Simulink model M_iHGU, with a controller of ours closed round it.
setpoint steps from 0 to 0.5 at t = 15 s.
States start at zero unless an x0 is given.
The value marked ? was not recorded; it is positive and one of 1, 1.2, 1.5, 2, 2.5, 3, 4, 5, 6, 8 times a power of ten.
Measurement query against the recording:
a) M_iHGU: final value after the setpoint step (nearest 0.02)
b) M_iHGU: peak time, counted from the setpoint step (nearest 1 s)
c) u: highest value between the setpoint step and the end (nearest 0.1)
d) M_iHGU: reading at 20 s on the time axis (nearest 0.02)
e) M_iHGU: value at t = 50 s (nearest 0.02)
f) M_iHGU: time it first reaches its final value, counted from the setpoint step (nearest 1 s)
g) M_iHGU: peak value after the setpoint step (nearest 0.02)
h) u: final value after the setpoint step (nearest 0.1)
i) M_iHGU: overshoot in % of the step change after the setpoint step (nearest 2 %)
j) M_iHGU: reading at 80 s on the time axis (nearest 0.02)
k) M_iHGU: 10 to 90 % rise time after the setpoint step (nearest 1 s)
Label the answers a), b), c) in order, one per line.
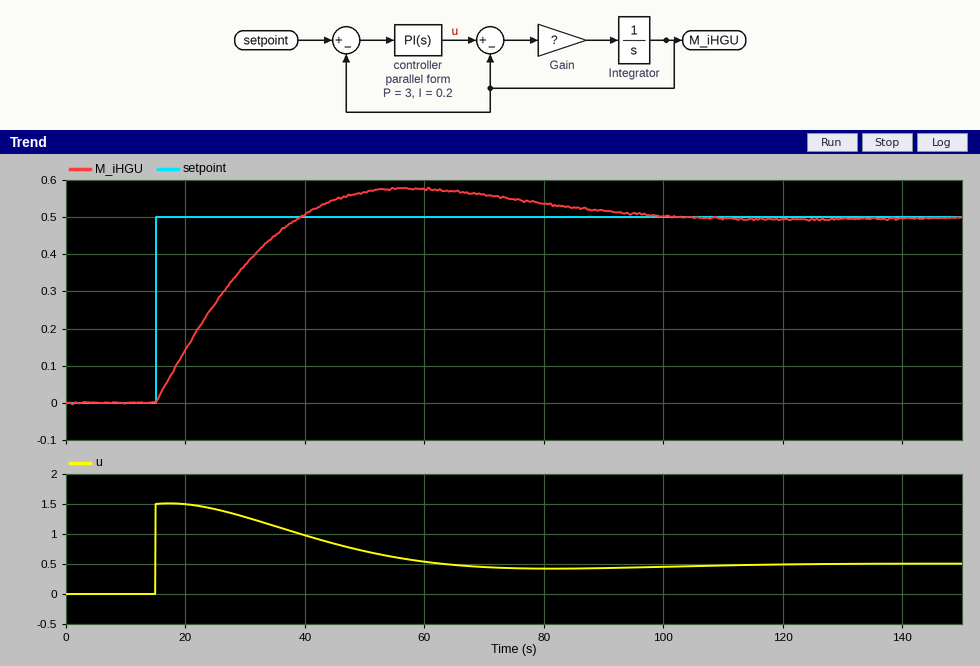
a) 0.50
b) 42 s
c) 1.5
d) 0.14
e) 0.56
f) 24 s
g) 0.58
h) 0.5
i) 16 %
j) 0.54
k) 18 s
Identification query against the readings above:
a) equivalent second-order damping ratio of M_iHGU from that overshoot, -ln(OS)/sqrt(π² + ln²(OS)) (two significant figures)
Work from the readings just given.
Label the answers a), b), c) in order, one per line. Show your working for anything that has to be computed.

a) ln(0.16) = -1.833; 1.833 / sqrt(9.870 + 3.358) = 0.50
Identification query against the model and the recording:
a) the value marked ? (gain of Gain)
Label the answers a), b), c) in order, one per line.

a) 0.02
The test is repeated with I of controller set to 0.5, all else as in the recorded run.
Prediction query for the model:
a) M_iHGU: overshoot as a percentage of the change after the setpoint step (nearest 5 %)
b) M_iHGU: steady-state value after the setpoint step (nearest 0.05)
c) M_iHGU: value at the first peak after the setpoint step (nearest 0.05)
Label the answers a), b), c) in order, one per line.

a) 30 %
b) 0.50
c) 0.65
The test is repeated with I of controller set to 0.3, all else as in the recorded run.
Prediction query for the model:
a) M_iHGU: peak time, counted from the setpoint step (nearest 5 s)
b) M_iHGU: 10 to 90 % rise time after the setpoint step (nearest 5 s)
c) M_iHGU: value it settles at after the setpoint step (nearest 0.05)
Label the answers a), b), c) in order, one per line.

a) 35 s
b) 15 s
c) 0.50
